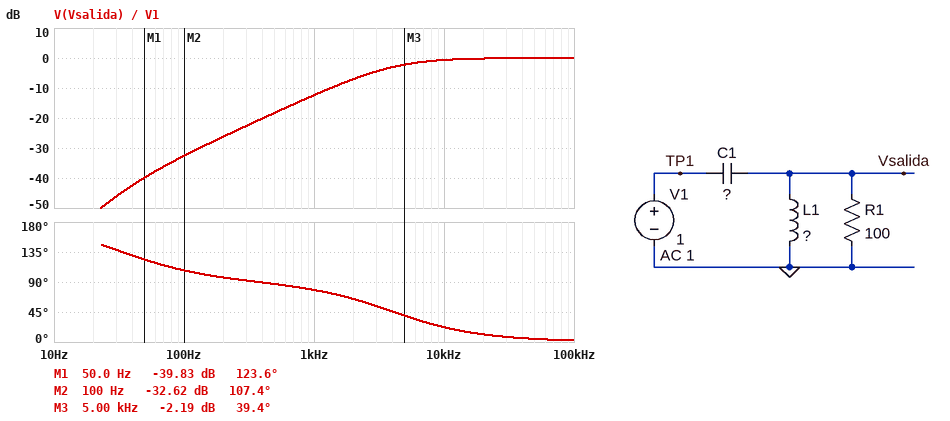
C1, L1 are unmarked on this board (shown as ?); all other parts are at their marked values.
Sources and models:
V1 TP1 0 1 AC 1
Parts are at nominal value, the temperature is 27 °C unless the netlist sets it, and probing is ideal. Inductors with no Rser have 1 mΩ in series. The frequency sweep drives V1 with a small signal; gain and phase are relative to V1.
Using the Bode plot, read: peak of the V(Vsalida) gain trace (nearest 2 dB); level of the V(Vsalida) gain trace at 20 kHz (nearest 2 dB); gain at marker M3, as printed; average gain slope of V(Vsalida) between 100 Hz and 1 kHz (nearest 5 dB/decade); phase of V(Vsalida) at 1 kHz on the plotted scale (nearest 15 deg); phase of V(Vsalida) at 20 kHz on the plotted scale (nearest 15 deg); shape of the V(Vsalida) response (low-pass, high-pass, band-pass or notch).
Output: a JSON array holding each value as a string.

["0 dB", "0 dB", "-2.19 dB", "20 dB/decade", "75 deg", "15 deg", "high-pass"]
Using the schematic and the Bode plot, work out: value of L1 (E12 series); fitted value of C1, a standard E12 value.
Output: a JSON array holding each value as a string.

["470 mH", "390 nF"]
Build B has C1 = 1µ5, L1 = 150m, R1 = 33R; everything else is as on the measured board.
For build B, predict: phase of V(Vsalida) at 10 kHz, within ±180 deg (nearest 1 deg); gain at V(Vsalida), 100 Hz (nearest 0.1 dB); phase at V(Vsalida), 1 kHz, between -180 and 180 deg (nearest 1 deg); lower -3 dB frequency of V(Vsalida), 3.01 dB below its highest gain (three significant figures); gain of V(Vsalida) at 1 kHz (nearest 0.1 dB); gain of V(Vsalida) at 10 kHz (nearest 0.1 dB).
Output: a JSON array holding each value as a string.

["18 deg", "-30.6 dB", "75 deg", "3.18 kHz", "-10.5 dB", "-0.4 dB"]
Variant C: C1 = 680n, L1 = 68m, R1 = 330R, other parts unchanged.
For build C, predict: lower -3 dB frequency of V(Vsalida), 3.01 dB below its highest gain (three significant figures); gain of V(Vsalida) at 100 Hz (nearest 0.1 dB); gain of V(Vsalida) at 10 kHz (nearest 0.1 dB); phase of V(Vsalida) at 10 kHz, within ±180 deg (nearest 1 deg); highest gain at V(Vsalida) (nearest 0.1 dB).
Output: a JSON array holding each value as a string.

["630 Hz", "-34.7 dB", "0 dB", "4 deg", "1.5 dB"]
